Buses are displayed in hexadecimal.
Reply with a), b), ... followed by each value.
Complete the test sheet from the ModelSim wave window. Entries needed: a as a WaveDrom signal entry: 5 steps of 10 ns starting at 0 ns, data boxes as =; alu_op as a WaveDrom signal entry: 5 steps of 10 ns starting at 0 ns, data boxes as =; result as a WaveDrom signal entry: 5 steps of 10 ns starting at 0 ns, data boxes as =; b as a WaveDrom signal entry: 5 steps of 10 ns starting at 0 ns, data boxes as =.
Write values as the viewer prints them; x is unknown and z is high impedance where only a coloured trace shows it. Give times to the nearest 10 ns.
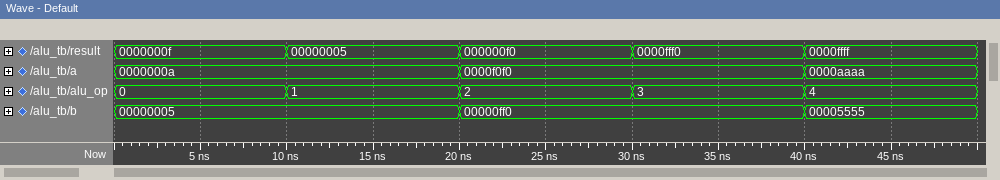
a) {name: 'a', wave: '=.=.=', data: '0000000a 0000f0f0 0000aaaa'}
b) {name: 'alu_op', wave: '=====', data: '0 1 2 3 4'}
c) {name: 'result', wave: '=====', data: '0000000f 00000005 000000f0 0000fff0 0000ffff'}
d) {name: 'b', wave: '=.=.=', data: '00000005 00000ff0 00005555'}
